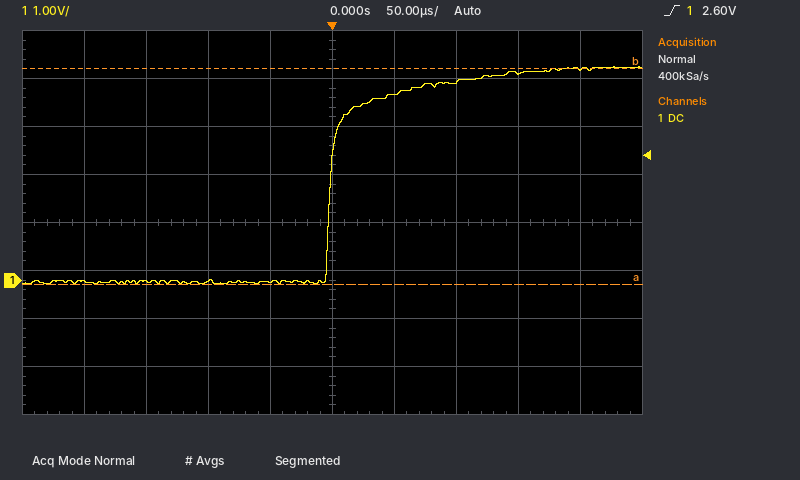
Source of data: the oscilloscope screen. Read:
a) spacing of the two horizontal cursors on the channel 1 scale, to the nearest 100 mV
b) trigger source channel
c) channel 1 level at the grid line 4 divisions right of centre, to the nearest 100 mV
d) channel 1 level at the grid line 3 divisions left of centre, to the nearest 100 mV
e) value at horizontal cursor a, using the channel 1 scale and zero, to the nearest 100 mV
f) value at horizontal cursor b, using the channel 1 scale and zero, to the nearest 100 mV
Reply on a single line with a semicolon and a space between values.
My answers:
4.5 V; channel 1; 4.4 V; 0.0 V; -100 mV; 4.4 V
